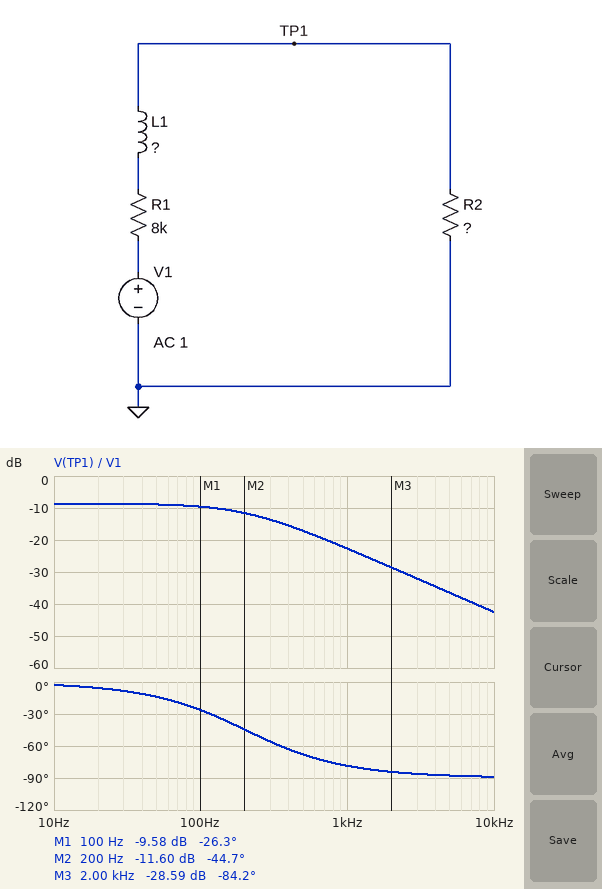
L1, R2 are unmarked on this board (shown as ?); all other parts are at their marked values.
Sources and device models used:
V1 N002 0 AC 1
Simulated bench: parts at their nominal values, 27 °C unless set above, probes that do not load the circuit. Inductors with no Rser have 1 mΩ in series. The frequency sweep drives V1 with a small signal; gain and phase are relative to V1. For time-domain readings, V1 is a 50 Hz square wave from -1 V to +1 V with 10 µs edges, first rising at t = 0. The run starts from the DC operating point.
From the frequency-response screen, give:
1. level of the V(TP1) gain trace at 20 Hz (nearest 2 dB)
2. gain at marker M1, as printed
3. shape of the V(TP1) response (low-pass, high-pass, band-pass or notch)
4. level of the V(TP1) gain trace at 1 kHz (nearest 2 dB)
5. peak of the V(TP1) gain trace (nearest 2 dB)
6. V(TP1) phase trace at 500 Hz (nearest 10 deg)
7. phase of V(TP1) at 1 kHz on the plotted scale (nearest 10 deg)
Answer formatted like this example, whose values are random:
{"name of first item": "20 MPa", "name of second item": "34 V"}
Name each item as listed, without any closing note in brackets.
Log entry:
{"level of the V(TP1) gain trace at 20 Hz": "-8 dB", "gain at marker M1, as printed": "-9.58 dB", "shape of the V(TP1) response": "low-pass", "level of the V(TP1) gain trace at 1 kHz": "-22 dB", "peak of the V(TP1) gain trace": "-8 dB", "V(TP1) phase trace at 500 Hz": "-70 deg", "phase of V(TP1) at 1 kHz on the plotted scale": "-80 deg"}
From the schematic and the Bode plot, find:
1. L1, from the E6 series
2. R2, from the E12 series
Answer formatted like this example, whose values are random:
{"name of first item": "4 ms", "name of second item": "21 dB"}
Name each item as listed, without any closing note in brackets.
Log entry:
{"L1, from the E6 series": "10 H", "R2, from the E12 series": "4.7 kΩ"}
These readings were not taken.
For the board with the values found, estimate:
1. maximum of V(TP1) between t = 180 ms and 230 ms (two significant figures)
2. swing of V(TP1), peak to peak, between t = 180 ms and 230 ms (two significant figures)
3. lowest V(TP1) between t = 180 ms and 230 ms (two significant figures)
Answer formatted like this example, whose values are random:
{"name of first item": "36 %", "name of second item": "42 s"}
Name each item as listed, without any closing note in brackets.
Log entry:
{"maximum of V(TP1) between t = 180 ms and 230 ms": "370 mV", "swing of V(TP1), peak to peak, between t = 180 ms and 230 ms": "740 mV", "lowest V(TP1) between t = 180 ms and 230 ms": "-370 mV"}
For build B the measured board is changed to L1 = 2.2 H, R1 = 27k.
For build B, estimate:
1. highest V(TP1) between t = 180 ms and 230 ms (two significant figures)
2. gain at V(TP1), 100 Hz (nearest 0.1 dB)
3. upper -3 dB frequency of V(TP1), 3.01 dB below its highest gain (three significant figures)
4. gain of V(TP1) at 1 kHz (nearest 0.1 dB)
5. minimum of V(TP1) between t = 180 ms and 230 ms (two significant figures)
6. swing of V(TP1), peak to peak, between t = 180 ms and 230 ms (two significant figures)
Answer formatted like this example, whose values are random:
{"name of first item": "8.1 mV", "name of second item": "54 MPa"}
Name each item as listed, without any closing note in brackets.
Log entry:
{"highest V(TP1) between t = 180 ms and 230 ms": "150 mV", "gain at V(TP1), 100 Hz": "-16.6 dB", "upper -3 dB frequency of V(TP1), 3.01 dB below its highest gain": "2.29 kHz", "gain of V(TP1) at 1 kHz": "-17.3 dB", "minimum of V(TP1) between t = 180 ms and 230 ms": "-150 mV", "swing of V(TP1), peak to peak, between t = 180 ms and 230 ms": "300 mV"}
